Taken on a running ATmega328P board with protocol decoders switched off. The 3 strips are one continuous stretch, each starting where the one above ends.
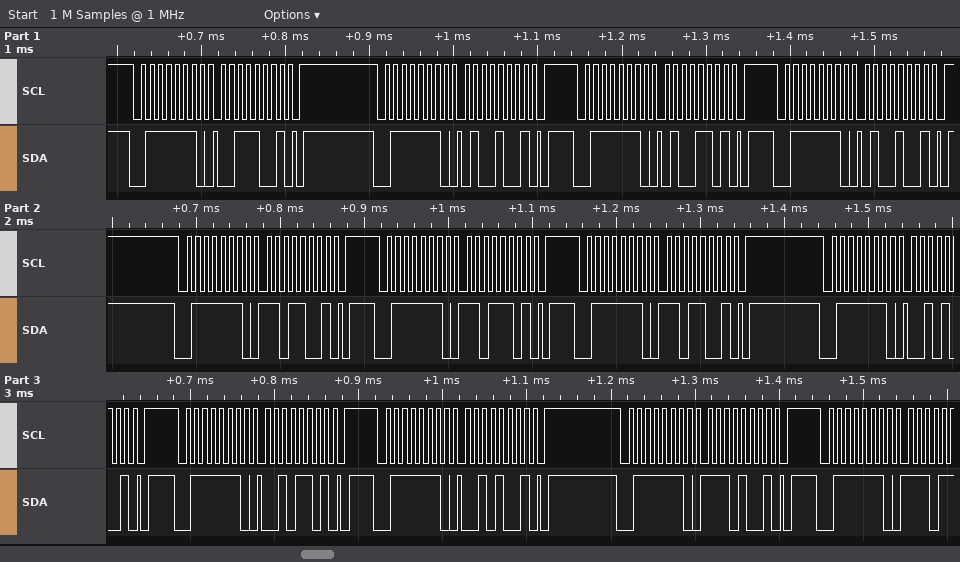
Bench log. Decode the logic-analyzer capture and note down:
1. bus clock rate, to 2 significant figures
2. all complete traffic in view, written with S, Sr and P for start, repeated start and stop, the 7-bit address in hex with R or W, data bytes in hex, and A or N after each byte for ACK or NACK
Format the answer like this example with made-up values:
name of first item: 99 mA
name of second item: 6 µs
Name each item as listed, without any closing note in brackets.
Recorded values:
bus clock rate, to 2 significant figures: 100 kHz
all complete traffic in view, written with S, Sr and P for start, repeated start and stop, the 7-bit address in hex with R or W, data bytes in hex, and A or N after each byte for ACK or NACK: S 3FW A 39 A P S 3FW A 49 A P S 3FW A 4D A P S 3FW A 49 A P S 3FW A D9 A P S 3FW A DD A P S 3FW A D9 A P S 3FW A 29 A P S 3FW A 2D A P S 3FW A 29 A P S 3FW A E9 A P S 3FW A
